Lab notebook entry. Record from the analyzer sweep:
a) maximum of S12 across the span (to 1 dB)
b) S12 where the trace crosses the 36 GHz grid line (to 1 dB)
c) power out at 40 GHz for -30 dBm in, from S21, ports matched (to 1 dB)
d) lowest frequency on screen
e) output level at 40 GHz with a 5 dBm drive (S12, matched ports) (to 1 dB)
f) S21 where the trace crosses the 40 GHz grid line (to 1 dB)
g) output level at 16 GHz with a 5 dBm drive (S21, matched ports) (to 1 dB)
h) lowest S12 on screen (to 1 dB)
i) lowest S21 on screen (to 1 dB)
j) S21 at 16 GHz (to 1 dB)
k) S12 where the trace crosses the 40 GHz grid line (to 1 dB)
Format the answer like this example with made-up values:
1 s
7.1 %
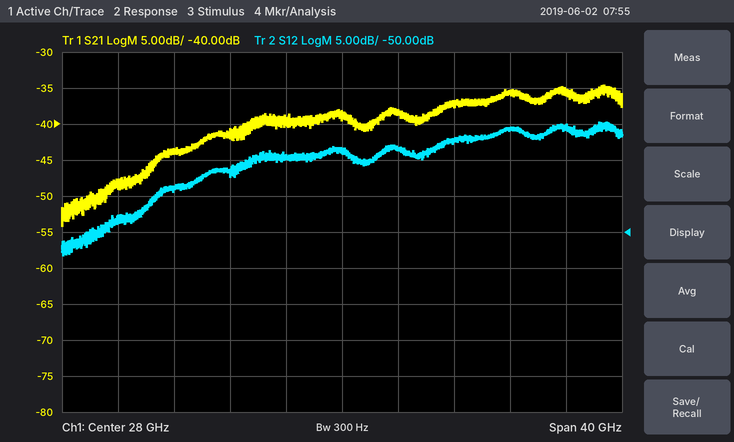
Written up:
-35 dB
-37 dB
-66 dBm
8 GHz
-31 dBm
-36 dB
-39 dBm
-53 dB
-54 dB
-44 dB
-36 dB
